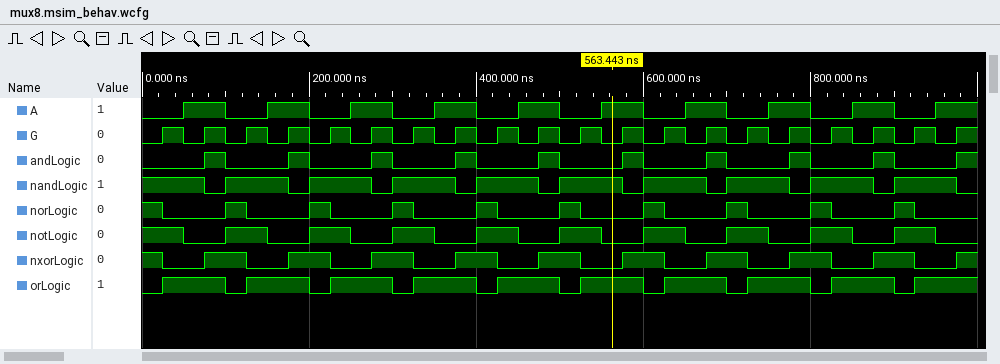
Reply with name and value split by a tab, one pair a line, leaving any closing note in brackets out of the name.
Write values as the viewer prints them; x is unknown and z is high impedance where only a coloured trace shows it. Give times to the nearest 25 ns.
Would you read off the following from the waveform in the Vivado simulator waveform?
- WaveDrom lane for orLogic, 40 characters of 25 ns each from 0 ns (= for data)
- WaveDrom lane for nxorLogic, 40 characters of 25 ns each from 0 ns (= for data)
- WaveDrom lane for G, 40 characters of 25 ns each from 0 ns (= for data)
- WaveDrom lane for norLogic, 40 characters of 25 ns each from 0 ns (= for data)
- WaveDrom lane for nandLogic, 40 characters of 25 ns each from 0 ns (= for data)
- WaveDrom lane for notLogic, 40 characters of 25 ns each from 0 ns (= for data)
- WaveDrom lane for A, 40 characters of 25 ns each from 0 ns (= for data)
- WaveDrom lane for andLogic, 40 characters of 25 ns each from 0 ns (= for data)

WaveDrom lane for orLogic, 40 characters of 25 ns each from 0 ns	{name: 'orLogic', wave: '01..01..01..01..01..01..01..01..01..01..'}
WaveDrom lane for nxorLogic, 40 characters of 25 ns each from 0 ns	{name: 'nxorLogic', wave: '10.1.0.1.0.1.0.1.0.1.0.1.0.1.0.1.0.1.0.1'}
WaveDrom lane for G, 40 characters of 25 ns each from 0 ns	{name: 'G', wave: '0101010101010101010101010101010101010101'}
WaveDrom lane for norLogic, 40 characters of 25 ns each from 0 ns	{name: 'norLogic', wave: '10..10..10..10..10..10..10..10..10..10..'}
WaveDrom lane for nandLogic, 40 characters of 25 ns each from 0 ns	{name: 'nandLogic', wave: '1..01..01..01..01..01..01..01..01..01..0'}
WaveDrom lane for notLogic, 40 characters of 25 ns each from 0 ns	{name: 'notLogic', wave: '1.0.1.0.1.0.1.0.1.0.1.0.1.0.1.0.1.0.1.0.'}
WaveDrom lane for A, 40 characters of 25 ns each from 0 ns	{name: 'A', wave: '0.1.0.1.0.1.0.1.0.1.0.1.0.1.0.1.0.1.0.1.'}
WaveDrom lane for andLogic, 40 characters of 25 ns each from 0 ns	{name: 'andLogic', wave: '0..10..10..10..10..10..10..10..10..10..1'}
